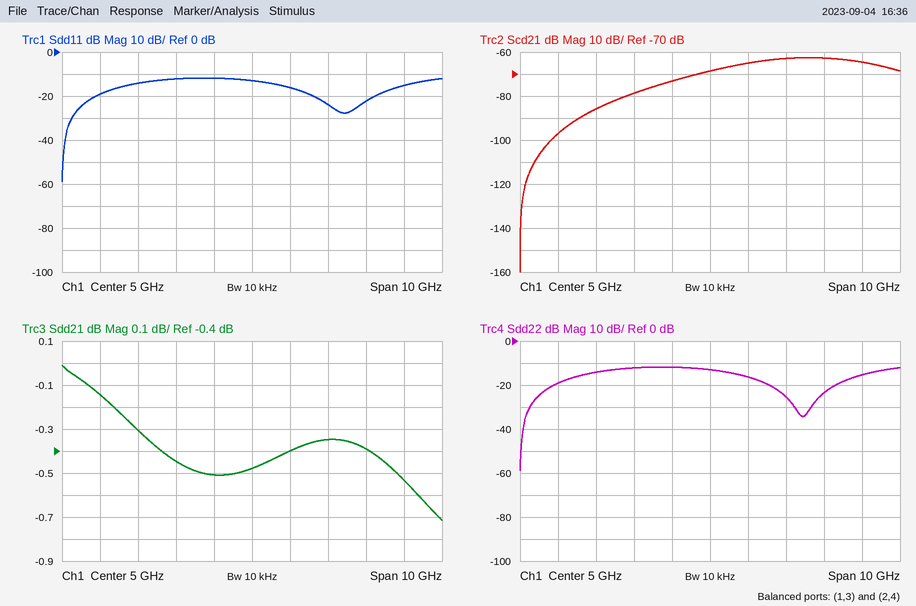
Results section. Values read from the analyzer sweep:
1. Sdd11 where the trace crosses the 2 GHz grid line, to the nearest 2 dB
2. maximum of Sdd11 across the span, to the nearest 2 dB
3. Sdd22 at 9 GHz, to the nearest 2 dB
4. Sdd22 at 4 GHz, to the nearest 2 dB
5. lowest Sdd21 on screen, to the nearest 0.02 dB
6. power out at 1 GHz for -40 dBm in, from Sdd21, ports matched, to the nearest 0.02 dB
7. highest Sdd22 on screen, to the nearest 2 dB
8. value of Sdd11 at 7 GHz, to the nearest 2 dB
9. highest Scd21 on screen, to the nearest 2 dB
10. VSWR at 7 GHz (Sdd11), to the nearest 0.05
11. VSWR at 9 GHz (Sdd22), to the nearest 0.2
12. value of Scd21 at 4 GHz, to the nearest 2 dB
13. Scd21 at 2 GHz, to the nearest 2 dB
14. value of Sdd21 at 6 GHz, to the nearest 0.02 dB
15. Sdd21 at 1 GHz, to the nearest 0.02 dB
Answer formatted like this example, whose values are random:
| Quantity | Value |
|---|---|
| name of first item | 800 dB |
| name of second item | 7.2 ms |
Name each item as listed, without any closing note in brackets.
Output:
| Quantity | Value |
|---|---|
| Sdd11 where the trace crosses the 2 GHz grid line, to the nearest 2 dB | -14 dB |
| maximum of Sdd11 across the span, to the nearest 2 dB | -12 dB |
| Sdd22 at 9 GHz, to the nearest 2 dB | -16 dB |
| Sdd22 at 4 GHz, to the nearest 2 dB | -12 dB |
| lowest Sdd21 on screen, to the nearest 0.02 dB | -0.72 dB |
| power out at 1 GHz for -40 dBm in, from Sdd21, ports matched, to the nearest 0.02 dB | -40.14 dBm |
| highest Sdd22 on screen, to the nearest 2 dB | -12 dB |
| value of Sdd11 at 7 GHz, to the nearest 2 dB | -24 dB |
| highest Scd21 on screen, to the nearest 2 dB | -62 dB |
| VSWR at 7 GHz (Sdd11), to the nearest 0.05 | 1.15 |
| VSWR at 9 GHz (Sdd22), to the nearest 0.2 | 1.4 |
| value of Scd21 at 4 GHz, to the nearest 2 dB | -74 dB |
| Scd21 at 2 GHz, to the nearest 2 dB | -86 dB |
| value of Sdd21 at 6 GHz, to the nearest 0.02 dB | -0.40 dB |
| Sdd21 at 1 GHz, to the nearest 0.02 dB | -0.14 dB |
